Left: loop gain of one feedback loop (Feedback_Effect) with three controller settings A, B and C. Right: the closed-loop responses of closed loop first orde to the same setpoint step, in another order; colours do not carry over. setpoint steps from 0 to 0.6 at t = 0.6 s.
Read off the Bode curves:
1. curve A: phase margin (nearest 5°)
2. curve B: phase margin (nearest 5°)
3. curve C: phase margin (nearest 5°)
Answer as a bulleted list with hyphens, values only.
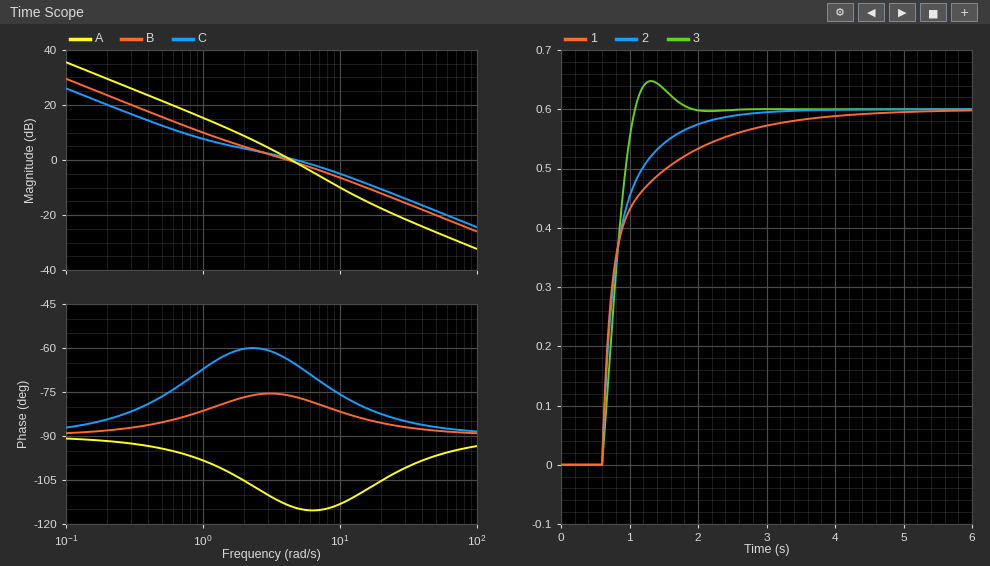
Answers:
- 65°
- 105°
- 115°
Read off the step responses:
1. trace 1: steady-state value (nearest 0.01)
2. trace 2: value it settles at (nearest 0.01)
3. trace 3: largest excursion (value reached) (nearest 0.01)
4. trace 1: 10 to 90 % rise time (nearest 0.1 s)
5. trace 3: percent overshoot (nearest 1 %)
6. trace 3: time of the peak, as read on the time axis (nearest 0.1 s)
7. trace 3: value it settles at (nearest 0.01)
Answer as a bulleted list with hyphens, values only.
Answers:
- 0.60
- 0.60
- 0.65
- 1.5 s
- 8 %
- 1.3 s
- 0.60
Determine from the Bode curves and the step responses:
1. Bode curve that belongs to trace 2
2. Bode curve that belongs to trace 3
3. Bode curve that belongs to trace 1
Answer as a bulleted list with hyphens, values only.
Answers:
- B
- A
- C
